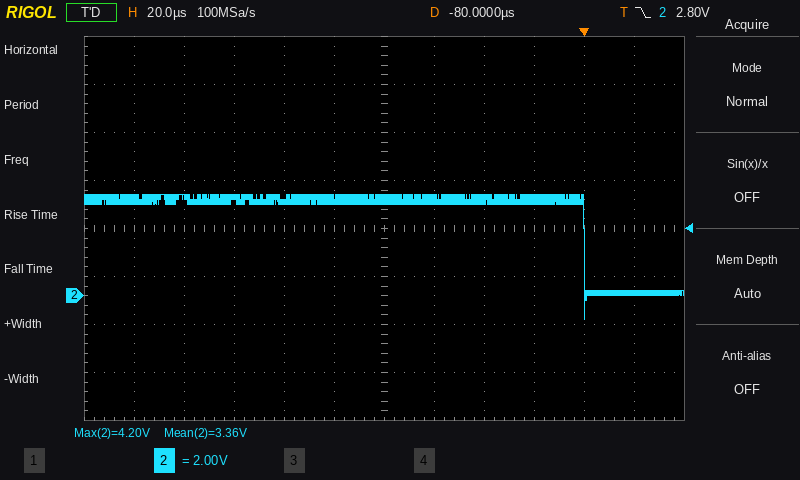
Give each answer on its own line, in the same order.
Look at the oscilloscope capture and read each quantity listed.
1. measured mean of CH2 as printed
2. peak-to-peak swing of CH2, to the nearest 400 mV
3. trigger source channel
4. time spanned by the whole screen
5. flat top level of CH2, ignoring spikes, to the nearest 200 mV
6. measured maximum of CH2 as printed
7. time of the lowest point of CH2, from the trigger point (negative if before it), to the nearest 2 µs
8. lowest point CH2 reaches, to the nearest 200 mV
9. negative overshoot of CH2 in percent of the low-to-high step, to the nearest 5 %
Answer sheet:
3.36 V
5.2 V
CH2
240 µs
4.0 V
4.20 V
0 µs
-1.0 V
30 %
